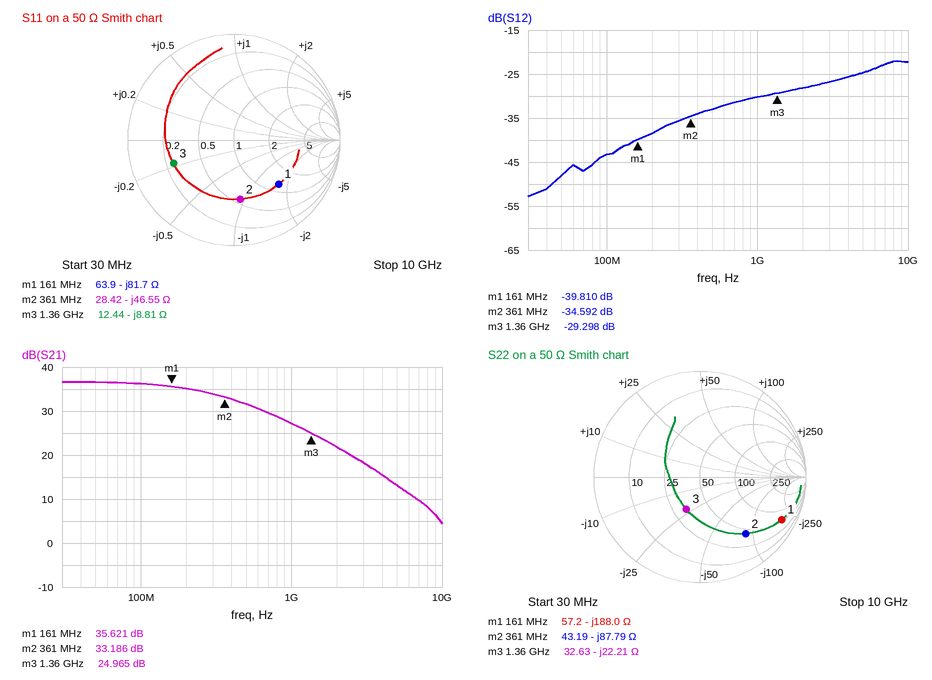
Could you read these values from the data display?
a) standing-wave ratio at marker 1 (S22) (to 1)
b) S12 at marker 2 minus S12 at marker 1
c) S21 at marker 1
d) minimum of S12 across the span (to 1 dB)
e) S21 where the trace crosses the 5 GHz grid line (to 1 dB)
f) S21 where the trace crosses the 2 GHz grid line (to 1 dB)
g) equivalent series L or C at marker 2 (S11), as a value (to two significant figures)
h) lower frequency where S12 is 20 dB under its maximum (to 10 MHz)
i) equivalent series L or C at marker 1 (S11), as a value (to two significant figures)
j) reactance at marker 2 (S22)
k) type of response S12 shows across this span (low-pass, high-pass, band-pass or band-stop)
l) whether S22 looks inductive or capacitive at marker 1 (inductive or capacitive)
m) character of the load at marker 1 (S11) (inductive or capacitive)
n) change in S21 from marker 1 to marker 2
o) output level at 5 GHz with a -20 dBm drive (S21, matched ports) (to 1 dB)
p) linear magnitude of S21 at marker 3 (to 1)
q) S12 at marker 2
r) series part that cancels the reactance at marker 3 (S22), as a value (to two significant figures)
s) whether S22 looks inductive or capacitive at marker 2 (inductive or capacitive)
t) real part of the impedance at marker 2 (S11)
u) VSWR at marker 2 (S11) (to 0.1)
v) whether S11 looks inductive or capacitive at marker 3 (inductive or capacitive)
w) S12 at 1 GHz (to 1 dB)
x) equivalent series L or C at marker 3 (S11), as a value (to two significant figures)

14
5.218 dB
35.621 dB
-53 dB
13 dB
22 dB
9.5 pF
120 MHz
12 pF
-87.79 Ω
high-pass
capacitive
capacitive
-2.435 dB
-7 dBm
18
-34.592 dB
2.6 nH
capacitive
28.42 Ω
3.6
capacitive
-30 dB
13 pF
